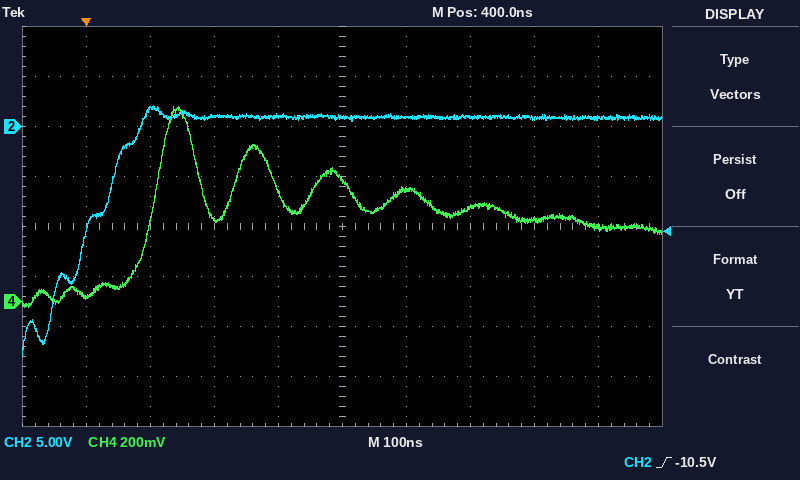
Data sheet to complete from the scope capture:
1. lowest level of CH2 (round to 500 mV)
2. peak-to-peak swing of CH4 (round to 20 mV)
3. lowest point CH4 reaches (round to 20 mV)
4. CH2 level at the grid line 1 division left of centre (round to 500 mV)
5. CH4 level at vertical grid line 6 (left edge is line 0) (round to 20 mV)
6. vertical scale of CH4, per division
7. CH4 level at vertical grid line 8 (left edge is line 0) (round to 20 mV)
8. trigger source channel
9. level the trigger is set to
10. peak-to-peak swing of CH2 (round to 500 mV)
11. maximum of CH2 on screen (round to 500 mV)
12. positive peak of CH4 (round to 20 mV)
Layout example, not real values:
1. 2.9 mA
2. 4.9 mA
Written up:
1. -23.0 V
2. 800 mV
3. -20 mV
4. 1.0 V
5. 440 mV
6. 200 mV
7. 320 mV
8. CH2
9. -10.5 V
10. 25.0 V
11. 2.0 V
12. 780 mV
